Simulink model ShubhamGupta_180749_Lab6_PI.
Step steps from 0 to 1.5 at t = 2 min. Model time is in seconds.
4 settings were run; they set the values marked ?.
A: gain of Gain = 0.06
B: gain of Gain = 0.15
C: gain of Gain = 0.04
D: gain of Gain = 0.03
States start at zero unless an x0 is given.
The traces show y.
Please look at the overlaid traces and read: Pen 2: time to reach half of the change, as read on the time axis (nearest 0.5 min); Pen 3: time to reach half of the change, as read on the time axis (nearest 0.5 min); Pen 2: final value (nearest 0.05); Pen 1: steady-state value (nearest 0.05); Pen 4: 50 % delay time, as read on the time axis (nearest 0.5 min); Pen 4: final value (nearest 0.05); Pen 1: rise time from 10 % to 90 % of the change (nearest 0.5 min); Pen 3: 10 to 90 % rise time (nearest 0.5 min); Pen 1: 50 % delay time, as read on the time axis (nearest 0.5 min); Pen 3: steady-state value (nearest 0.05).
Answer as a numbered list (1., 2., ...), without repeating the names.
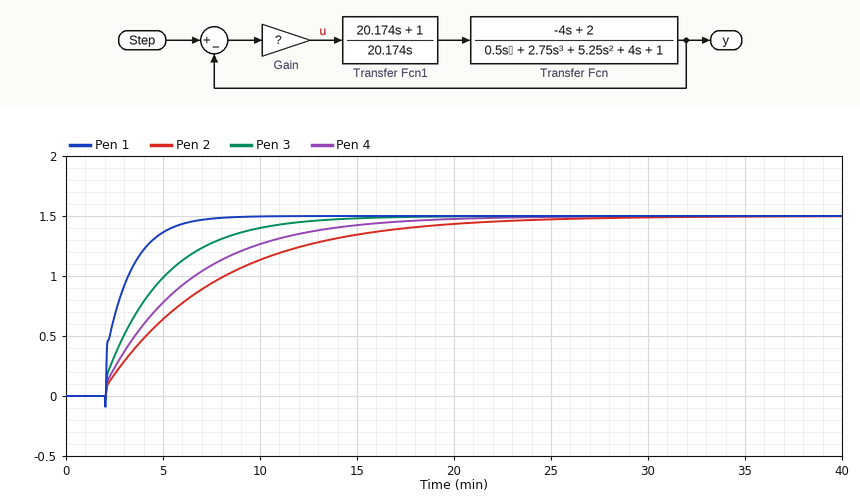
1. 6.0 min
2. 4.0 min
3. 1.50
4. 1.50
5. 5.0 min
6. 1.50
7. 3.0 min
8. 6.5 min
9. 2.5 min
10. 1.50
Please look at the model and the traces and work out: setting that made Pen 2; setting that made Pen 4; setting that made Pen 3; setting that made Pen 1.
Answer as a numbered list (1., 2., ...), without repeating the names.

1. D
2. C
3. A
4. B
